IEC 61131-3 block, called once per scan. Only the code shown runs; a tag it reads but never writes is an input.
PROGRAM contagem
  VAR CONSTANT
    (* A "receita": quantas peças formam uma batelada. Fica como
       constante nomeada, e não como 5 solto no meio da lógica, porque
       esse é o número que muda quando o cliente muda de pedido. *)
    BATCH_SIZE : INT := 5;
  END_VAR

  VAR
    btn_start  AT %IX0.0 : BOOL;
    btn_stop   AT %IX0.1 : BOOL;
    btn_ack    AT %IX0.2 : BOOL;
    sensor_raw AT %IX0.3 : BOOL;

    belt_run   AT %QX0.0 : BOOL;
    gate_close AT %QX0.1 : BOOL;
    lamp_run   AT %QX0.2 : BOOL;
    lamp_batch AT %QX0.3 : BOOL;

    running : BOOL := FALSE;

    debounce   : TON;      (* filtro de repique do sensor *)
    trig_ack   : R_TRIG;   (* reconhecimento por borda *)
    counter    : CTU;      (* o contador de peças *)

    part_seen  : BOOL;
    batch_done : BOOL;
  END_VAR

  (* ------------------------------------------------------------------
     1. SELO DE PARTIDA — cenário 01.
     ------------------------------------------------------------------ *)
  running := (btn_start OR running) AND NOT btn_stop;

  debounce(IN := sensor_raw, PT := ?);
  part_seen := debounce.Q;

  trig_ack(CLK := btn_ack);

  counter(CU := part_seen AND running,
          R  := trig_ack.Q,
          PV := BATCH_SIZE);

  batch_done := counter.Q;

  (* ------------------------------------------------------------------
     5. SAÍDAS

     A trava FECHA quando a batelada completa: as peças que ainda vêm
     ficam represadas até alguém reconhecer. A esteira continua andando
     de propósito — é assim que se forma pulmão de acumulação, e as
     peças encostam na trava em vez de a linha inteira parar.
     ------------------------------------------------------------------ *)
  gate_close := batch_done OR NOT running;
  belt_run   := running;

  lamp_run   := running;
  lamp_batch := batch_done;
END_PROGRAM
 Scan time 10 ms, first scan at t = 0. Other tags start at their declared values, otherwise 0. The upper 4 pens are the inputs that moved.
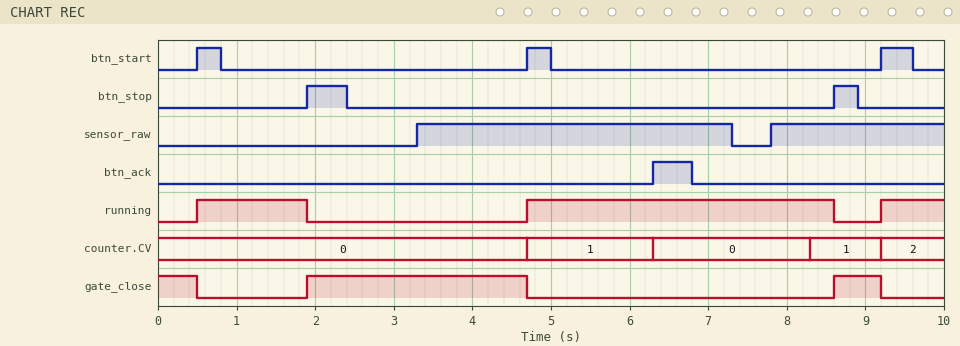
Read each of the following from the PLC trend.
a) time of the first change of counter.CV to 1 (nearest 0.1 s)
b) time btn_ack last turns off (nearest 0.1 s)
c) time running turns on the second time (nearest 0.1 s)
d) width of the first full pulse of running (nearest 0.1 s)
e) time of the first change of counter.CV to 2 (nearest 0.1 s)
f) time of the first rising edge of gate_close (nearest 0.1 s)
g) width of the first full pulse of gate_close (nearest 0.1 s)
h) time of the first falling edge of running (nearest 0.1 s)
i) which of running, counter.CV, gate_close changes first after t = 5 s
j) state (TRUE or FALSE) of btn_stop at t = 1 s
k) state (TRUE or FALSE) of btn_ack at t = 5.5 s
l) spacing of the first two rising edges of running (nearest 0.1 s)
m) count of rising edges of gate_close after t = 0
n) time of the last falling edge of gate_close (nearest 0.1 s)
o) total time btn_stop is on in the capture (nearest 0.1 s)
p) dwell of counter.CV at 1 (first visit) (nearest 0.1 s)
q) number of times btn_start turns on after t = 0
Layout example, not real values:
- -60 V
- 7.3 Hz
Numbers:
- 4.7 s
- 6.8 s
- 4.7 s
- 1.4 s
- 9.2 s
- 1.9 s
- 2.8 s
- 1.9 s
- counter.CV
- FALSE
- FALSE
- 4.2 s
- 2
- 9.2 s
- 0.8 s
- 1.6 s
- 3
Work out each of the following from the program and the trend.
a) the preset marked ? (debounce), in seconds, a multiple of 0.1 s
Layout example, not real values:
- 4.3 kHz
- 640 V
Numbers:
- 0.5 s
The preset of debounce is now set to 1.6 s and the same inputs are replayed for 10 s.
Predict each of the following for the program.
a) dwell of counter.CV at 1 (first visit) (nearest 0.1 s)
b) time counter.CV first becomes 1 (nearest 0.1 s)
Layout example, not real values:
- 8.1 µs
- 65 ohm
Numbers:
- 1.4 s
- 4.9 s
